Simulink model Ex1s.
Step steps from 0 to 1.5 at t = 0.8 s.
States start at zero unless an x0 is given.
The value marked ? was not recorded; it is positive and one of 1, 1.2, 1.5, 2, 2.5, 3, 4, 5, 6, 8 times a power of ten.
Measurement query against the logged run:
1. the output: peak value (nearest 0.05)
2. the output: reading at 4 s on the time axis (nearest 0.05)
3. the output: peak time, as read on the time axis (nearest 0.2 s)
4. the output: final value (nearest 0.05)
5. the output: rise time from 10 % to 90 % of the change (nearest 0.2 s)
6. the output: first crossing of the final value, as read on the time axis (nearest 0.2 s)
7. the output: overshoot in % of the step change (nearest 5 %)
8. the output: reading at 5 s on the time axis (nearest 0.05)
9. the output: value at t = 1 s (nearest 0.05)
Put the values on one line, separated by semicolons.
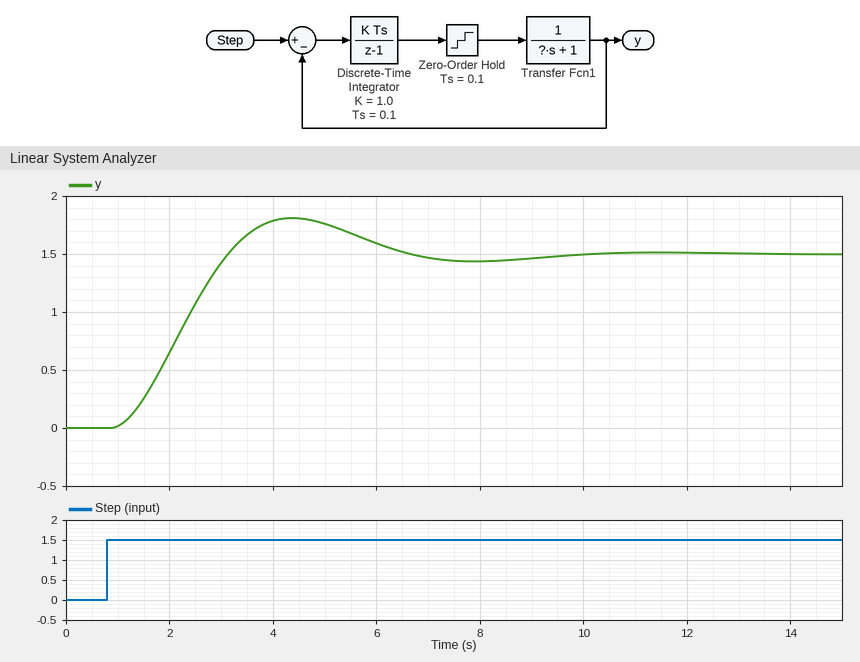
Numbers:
1.80; 1.80; 4.4 s; 1.50; 1.6 s; 3.2 s; 20 %; 1.75; 0.00
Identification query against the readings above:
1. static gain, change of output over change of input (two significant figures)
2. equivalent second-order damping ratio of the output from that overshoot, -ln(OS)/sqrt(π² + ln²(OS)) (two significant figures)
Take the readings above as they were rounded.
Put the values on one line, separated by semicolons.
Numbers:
1.0; 0.46
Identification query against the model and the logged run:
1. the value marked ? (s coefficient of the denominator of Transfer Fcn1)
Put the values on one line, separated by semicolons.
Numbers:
1
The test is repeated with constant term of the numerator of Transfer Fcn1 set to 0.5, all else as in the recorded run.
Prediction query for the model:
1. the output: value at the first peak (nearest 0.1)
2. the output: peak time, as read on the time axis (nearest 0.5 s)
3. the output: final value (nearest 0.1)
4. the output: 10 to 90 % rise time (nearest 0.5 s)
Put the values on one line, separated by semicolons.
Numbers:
1.6; 7.0 s; 1.5; 3.0 s
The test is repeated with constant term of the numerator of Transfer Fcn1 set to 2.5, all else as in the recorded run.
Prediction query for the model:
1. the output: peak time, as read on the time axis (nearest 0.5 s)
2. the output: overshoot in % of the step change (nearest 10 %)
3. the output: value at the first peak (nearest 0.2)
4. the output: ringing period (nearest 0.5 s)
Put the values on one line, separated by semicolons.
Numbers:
3.0 s; 50 %; 2.2; 4.0 s
